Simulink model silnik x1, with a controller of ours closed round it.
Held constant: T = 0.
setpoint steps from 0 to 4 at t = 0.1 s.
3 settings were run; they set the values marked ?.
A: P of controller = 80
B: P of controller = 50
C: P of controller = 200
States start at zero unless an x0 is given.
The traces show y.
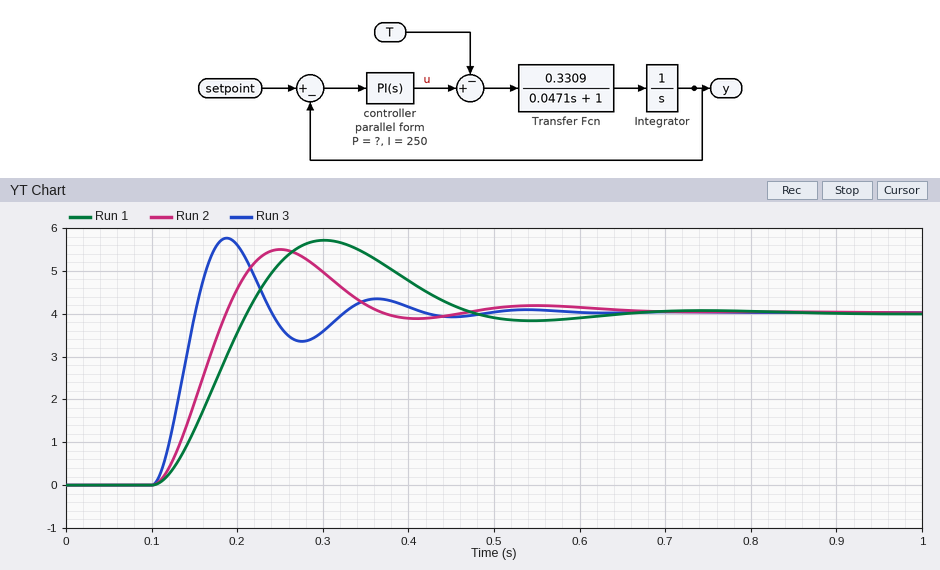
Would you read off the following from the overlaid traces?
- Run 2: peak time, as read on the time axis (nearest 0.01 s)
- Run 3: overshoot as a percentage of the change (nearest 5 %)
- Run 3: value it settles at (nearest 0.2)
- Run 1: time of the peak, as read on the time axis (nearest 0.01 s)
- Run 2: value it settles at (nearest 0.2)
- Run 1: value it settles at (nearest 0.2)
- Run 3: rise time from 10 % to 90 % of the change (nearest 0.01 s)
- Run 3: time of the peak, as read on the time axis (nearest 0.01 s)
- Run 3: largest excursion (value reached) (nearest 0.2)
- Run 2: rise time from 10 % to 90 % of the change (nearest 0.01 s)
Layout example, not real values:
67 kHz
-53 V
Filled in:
0.25 s
45 %
4.0
0.30 s
4.0
4.0
0.03 s
0.19 s
5.8
0.06 s
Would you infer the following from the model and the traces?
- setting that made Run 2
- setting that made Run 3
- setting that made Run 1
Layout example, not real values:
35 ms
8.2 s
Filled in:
A
C
B
